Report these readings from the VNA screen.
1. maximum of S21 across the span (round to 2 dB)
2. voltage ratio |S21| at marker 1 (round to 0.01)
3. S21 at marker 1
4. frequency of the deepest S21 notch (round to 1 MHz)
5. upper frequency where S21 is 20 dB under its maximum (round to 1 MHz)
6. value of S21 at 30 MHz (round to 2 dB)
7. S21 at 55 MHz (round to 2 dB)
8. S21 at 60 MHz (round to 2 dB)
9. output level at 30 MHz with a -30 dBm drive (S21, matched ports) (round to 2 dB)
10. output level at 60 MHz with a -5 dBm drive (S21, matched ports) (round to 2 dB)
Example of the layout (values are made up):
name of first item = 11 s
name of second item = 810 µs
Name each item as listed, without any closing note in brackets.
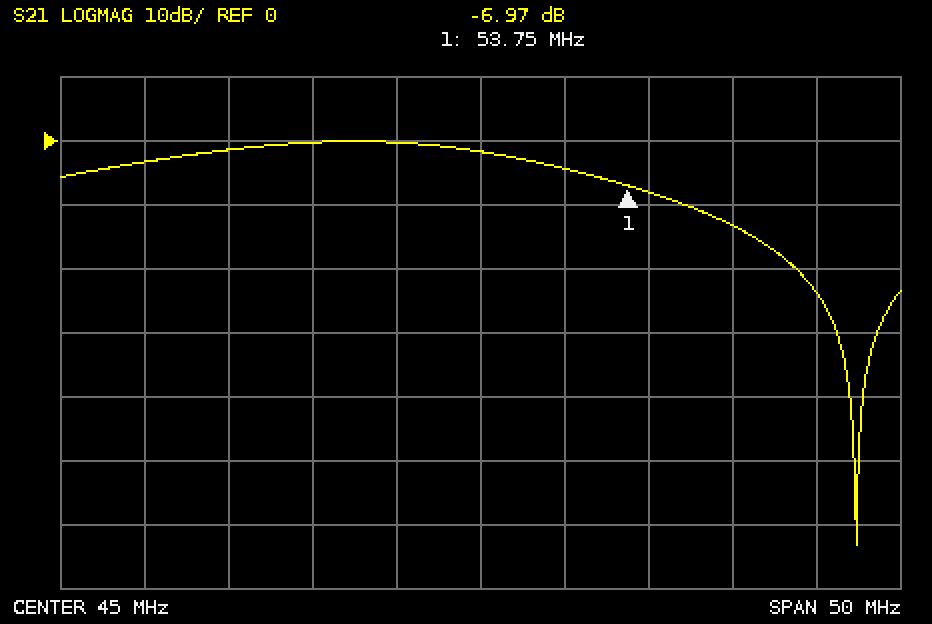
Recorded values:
maximum of S21 across the span = 0 dB
voltage ratio |S21| at marker 1 = 0.45
S21 at marker 1 = -6.97 dB
frequency of the deepest S21 notch = 67 MHz
upper frequency where S21 is 20 dB under its maximum = 64 MHz
value of S21 at 30 MHz = -2 dB
S21 at 55 MHz = -8 dB
S21 at 60 MHz = -14 dB
output level at 30 MHz with a -30 dBm drive (S21, matched ports) = -32 dBm
output level at 60 MHz with a -5 dBm drive (S21, matched ports) = -18 dBm
